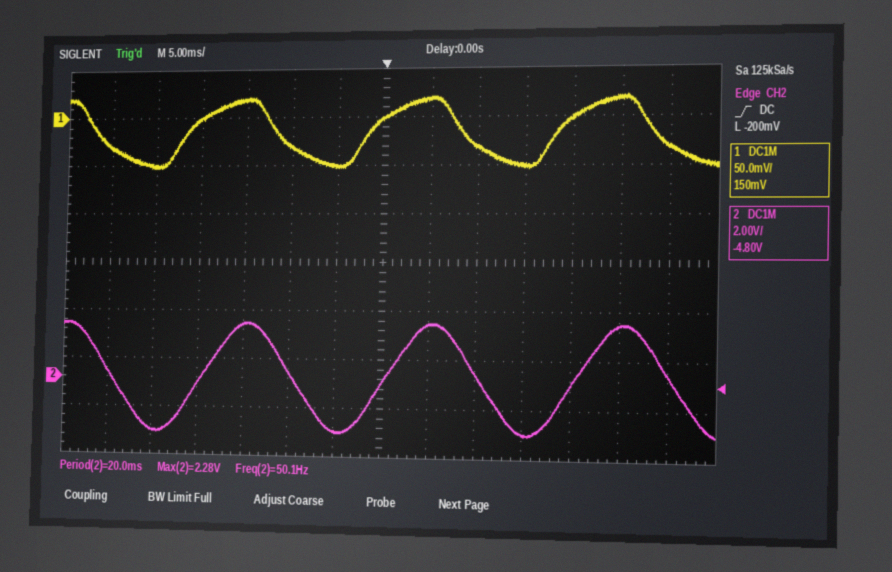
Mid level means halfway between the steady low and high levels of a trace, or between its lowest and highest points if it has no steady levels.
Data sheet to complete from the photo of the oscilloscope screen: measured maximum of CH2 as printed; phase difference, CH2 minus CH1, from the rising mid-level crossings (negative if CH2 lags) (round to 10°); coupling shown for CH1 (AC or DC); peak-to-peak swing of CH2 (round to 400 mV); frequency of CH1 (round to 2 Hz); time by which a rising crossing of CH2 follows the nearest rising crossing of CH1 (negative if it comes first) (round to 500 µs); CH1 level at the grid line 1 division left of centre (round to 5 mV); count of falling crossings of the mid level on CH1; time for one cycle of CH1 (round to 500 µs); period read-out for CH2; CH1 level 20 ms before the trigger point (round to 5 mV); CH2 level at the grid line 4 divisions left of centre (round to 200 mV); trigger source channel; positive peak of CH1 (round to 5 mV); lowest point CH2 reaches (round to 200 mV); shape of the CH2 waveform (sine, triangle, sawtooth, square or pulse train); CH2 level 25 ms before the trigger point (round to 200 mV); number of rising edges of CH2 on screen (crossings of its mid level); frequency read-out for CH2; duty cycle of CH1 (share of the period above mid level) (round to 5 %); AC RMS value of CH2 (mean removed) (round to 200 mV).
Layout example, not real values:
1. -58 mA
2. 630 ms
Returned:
1. 2.28 V
2. -40°
3. DC
4. 4.4 V
5. 50 Hz
6. +2.0 ms
7. -50 mV
8. 4
9. 20.0 ms
10. 20.0 ms
11. 0 mV
12. -200 mV
13. CH2
14. 20 mV
15. -2.2 V
16. sine
17. -2.2 V
18. 3
19. 50.1 Hz
20. 50 %
21. 1.6 V
